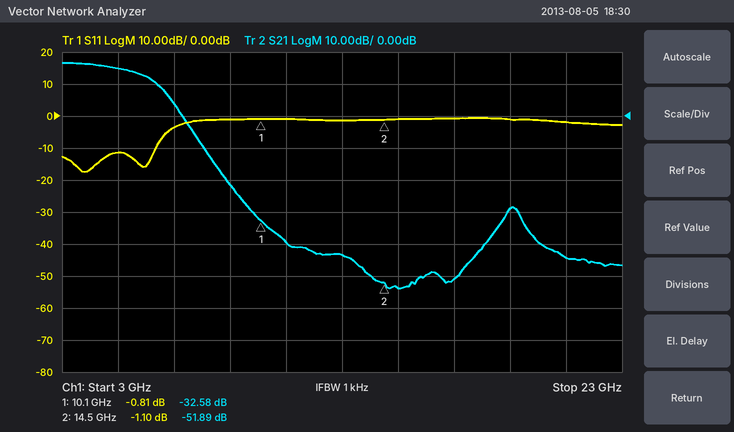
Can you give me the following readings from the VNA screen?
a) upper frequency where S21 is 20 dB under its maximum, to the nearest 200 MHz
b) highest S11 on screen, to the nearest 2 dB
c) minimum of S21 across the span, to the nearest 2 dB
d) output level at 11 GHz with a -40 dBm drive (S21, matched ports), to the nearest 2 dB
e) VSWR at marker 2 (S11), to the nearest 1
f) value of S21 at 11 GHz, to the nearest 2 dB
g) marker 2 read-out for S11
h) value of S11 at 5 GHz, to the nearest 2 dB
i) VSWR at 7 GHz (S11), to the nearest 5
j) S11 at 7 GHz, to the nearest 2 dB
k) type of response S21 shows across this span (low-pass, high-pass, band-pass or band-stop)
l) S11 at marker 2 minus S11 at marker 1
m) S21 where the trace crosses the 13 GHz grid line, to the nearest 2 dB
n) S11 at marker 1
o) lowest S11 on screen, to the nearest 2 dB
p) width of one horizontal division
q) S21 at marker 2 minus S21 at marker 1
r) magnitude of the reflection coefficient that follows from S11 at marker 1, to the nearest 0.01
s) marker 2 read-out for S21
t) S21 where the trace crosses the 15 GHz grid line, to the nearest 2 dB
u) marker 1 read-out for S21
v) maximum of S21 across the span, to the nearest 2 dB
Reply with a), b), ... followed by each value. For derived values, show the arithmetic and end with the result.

a) 7.6 GHz
b) 0 dB
c) -54 dB
d) -40 dBm + (-40 dB) = -80 dBm
e) (1 + 0.8810)/(1 − 0.8810) ≈ 16
f) -40 dB
g) -1.10 dB
h) -12 dB
i) |Γ| = 10^(-4/20) = 0.6310; VSWR = (1 + 0.6310)/(1 − 0.6310) ≈ 4.42, so 5 to the nearest 5
j) -4 dB
k) low-pass
l) -1.1 − (-0.81) = -0.29 dB
m) -44 dB
n) -0.81 dB
o) -18 dB
p) 2 GHz
q) -51.89 − (-32.58) = -19.31 dB
r) 10^(-0.81/20) ≈ 0.91
s) -51.89 dB
t) -54 dB
u) -32.58 dB
v) 16 dB
